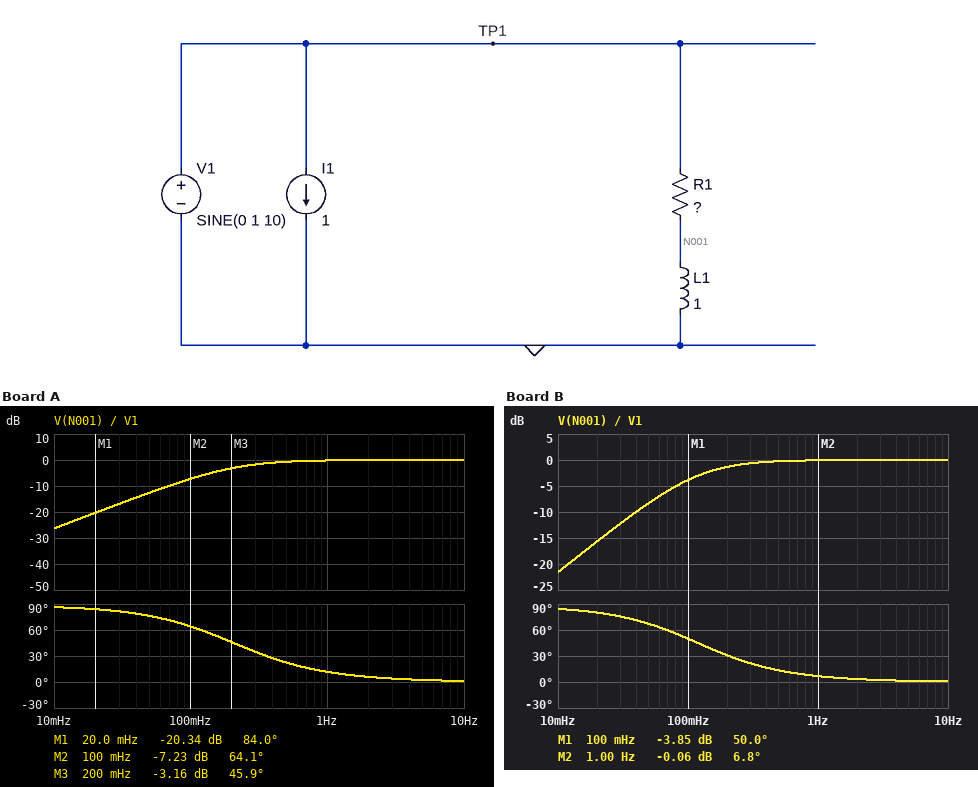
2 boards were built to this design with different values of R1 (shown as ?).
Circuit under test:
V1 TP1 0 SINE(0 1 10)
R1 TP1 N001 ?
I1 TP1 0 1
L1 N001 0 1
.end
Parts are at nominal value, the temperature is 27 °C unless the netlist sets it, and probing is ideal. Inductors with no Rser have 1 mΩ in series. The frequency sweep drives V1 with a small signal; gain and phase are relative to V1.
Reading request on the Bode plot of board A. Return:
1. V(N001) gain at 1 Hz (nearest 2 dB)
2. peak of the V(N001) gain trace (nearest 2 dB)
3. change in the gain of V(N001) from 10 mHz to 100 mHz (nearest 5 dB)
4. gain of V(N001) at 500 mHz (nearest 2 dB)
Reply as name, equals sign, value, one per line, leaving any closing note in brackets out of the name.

V(N001) gain at 1 Hz = 0 dB
peak of the V(N001) gain trace = 0 dB
change in the gain of V(N001) from 10 mHz to 100 mHz = 20 dB
gain of V(N001) at 500 mHz = 0 dB
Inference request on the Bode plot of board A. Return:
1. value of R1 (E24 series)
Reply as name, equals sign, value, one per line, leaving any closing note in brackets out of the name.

value of R1 = 1.3 Ω
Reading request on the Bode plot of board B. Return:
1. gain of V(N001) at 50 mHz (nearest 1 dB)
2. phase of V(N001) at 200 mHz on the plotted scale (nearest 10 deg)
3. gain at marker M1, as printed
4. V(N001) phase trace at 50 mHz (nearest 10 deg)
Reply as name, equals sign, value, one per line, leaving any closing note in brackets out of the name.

gain of V(N001) at 50 mHz = -8 dB
phase of V(N001) at 200 mHz on the plotted scale = 30 deg
gain at marker M1, as printed = -3.85 dB
V(N001) phase trace at 50 mHz = 70 deg
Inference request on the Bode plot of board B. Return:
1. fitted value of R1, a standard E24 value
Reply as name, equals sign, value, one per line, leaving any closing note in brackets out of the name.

fitted value of R1, a standard E24 value = 0.75 Ω
